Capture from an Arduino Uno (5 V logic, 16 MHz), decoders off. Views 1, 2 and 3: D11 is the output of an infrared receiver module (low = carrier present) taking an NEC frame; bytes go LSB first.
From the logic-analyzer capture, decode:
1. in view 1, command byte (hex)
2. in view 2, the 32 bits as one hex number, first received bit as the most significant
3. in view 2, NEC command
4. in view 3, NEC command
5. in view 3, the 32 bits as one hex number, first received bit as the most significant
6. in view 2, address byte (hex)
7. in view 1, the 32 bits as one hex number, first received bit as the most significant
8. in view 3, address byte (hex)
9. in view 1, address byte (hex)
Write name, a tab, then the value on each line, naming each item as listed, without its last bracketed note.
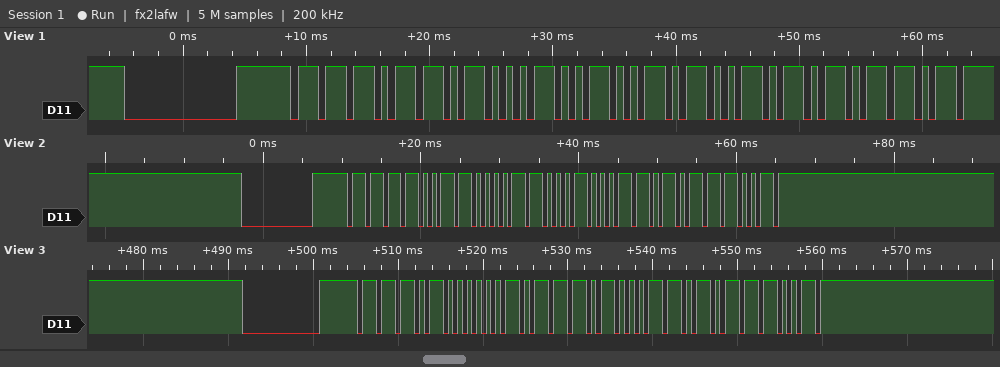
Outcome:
in view 1, command byte	0x4A
in view 2, the 32 bits as one hex number, first received bit as the most significant	0xF30C46B9
in view 2, NEC command	0x62
in view 3, NEC command	0x62
in view 3, the 32 bits as one hex number, first received bit as the most significant	0xE81746B9
in view 2, address byte	0xCF
in view 1, the 32 bits as one hex number, first received bit as the most significant	0xED1252AD
in view 3, address byte	0x17
in view 1, address byte	0xB7
